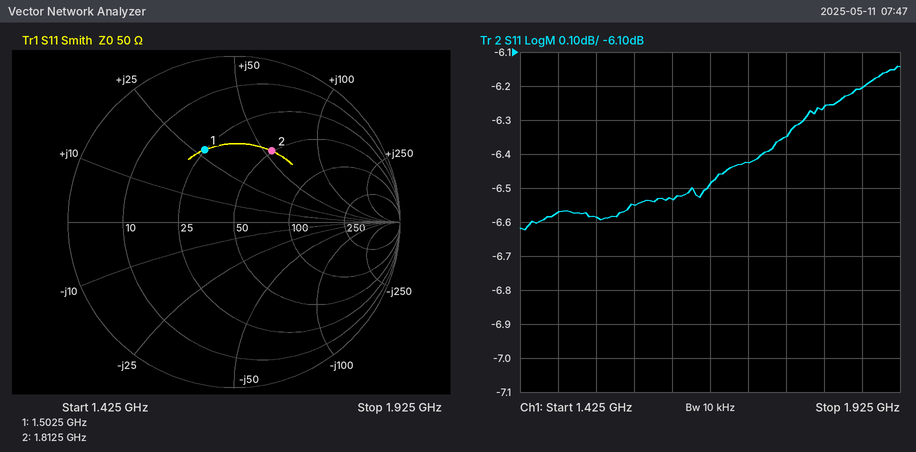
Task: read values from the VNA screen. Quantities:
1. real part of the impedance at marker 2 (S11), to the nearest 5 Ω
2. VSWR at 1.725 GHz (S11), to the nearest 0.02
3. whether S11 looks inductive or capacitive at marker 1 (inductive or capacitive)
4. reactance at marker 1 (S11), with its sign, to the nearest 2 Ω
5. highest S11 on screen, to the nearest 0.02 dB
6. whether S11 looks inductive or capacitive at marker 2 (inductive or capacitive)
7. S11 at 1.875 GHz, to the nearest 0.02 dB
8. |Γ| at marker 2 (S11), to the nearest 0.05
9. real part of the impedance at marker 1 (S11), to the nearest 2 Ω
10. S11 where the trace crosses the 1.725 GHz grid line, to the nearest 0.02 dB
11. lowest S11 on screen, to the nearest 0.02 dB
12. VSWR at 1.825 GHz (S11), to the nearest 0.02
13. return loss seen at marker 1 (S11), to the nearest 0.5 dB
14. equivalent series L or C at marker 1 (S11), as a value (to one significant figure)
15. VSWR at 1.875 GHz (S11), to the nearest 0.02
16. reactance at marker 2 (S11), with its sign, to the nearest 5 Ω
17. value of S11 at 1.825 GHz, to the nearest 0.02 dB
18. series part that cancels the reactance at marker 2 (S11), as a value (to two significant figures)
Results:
50 Ω
2.82
inductive
+28 Ω
-6.14 dB
inductive
-6.20 dB
0.50
24 Ω
-6.42 dB
-6.62 dB
2.90
6.5 dB
3 nH
2.92
+55 Ω
-6.26 dB
1.6 pF
